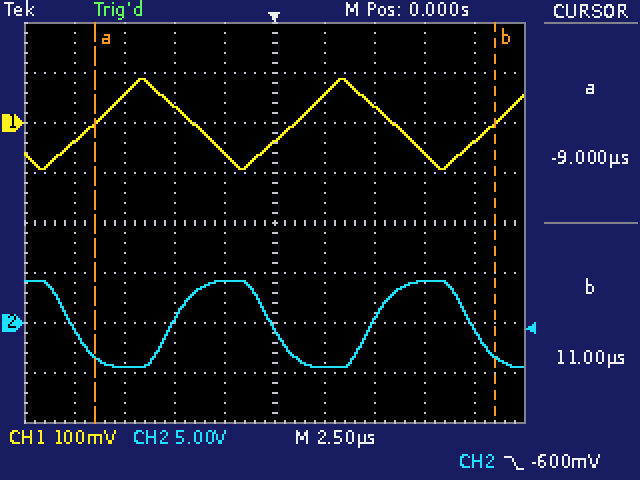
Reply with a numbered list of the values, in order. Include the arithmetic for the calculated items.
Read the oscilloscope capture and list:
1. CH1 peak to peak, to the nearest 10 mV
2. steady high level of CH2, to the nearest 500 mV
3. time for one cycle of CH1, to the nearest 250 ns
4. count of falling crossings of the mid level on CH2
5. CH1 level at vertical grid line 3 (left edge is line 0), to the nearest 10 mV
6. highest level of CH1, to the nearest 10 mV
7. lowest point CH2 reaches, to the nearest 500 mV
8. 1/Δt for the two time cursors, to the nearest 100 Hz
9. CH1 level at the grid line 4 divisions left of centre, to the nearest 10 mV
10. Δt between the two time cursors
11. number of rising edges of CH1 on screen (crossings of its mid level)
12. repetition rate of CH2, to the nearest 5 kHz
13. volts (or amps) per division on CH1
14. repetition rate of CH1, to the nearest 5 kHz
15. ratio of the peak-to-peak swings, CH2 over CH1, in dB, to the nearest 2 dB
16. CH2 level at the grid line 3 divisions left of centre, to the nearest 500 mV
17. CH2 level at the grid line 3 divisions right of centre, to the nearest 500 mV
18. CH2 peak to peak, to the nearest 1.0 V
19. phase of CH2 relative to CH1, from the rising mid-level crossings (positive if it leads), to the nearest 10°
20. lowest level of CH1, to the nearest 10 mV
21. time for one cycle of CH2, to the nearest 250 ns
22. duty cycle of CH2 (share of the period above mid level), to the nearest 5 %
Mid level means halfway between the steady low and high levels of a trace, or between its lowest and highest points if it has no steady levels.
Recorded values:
1. 90 mV − (-90 mV) = 180 mV
2. 4.0 V
3. 10.00 µs
4. 3
5. 30 mV
6. 90 mV
7. -4.5 V
8. 1 / 20.00 µs ≈ 50.0 kHz
9. -40 mV
10. 11 µs − (-9 µs) = 20.00 µs
11. 3
12. 1 / 10.00 µs ≈ 100 kHz
13. 100 mV
14. 1 / 10.00 µs ≈ 100 kHz
15. 20 log10(9.0 V / 180 mV) ≈ 34 dB
16. -4.5 V
17. 4.0 V
18. 9.0 V
19. -140°
20. -90 mV
21. 10.00 µs
22. 50 %
